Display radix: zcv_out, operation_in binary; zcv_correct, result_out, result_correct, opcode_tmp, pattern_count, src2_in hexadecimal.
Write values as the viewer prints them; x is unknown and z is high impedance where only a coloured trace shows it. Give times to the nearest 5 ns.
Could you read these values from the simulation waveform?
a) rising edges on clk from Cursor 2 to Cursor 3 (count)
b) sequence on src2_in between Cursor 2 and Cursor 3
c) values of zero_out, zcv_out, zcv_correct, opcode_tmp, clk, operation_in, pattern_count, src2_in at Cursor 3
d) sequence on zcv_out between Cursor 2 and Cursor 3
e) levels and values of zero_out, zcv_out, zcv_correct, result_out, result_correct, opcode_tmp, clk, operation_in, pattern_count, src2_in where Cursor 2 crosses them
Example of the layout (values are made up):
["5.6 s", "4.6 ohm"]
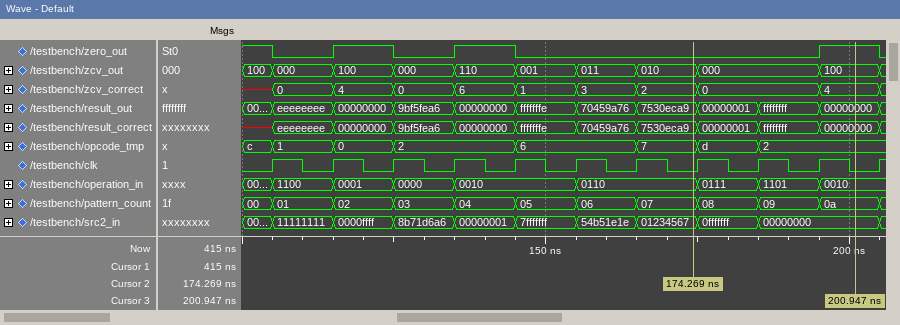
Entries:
["3", "01234567, 0fffffff, 00000000", "zero_out=1, zcv_out=100, zcv_correct=4, opcode_tmp=2, clk=0, operation_in=0010, pattern_count=0a, src2_in=00000000", "010, 000, 100", "zero_out=0, zcv_out=010, zcv_correct=2, result_out=7530eca9, result_correct=7530eca9, opcode_tmp=7, clk=0, operation_in=0110, pattern_count=07, src2_in=01234567"]
